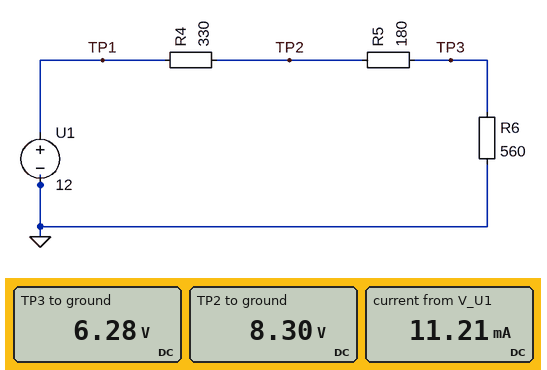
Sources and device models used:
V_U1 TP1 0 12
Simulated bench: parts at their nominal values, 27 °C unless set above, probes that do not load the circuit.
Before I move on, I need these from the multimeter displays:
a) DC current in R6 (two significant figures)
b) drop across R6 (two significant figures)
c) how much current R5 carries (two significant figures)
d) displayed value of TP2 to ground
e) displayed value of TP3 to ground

11 mA
6.3 V
11 mA
8.30 V
6.28 V
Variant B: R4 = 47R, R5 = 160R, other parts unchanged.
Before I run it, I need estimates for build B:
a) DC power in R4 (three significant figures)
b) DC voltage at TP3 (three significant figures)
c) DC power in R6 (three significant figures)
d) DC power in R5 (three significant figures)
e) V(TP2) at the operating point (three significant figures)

11.5 mW
8.76 V
137 mW
39.2 mW
11.3 V
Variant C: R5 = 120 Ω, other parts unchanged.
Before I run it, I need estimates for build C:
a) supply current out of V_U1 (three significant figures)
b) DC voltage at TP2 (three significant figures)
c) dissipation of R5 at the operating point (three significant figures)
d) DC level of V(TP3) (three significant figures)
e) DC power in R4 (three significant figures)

11.9 mA
8.08 V
16.9 mW
6.65 V
46.6 mW
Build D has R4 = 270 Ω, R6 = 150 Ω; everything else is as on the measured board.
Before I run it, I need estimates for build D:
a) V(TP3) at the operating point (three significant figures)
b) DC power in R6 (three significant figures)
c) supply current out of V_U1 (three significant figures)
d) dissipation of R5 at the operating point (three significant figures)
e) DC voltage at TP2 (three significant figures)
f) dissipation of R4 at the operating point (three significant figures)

3.00 V
60.0 mW
20.0 mA
72.0 mW
6.60 V
108 mW
